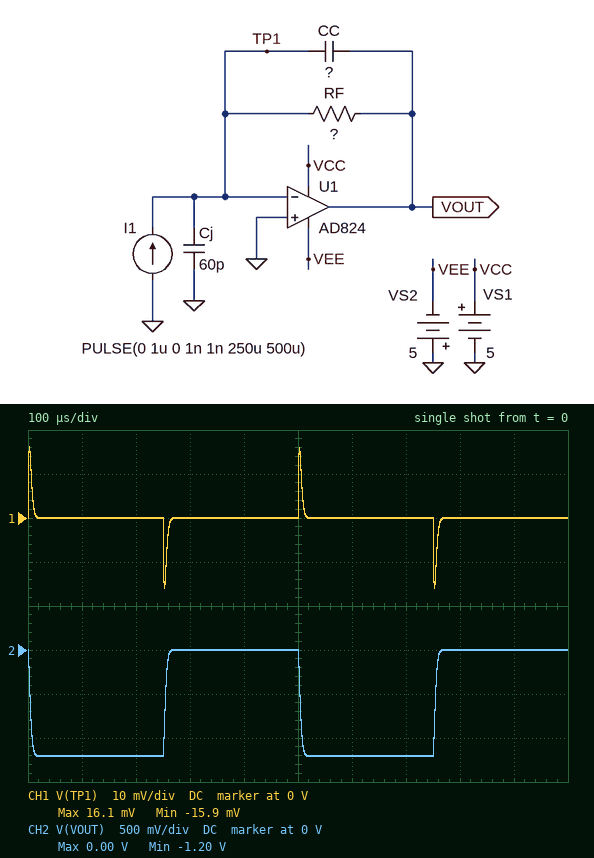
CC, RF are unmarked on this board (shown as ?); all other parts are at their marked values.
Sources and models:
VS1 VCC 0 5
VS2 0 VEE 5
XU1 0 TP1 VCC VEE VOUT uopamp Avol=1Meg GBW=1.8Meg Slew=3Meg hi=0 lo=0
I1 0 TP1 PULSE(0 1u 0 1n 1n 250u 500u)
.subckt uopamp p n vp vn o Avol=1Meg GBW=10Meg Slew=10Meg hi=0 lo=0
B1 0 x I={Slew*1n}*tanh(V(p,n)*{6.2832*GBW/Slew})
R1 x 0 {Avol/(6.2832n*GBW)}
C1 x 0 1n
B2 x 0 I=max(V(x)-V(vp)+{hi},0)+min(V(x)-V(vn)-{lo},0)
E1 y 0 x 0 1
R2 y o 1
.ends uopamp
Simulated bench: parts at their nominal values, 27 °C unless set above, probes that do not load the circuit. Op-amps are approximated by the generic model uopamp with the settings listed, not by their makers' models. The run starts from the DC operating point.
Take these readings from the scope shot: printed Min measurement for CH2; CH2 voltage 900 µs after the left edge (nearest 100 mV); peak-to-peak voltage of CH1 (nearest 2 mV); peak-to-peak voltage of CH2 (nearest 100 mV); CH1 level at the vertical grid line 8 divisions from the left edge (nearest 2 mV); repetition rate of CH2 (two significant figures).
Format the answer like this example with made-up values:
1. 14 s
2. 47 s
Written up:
1. -1.20 V
2. 0 V
3. 32 mV
4. 1.2 V
5. 0 V
6. 2.0 kHz
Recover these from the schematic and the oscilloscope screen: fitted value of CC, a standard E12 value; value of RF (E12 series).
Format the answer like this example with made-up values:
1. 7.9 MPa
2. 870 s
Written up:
1. 3.9 pF
2. 1.2 MΩ
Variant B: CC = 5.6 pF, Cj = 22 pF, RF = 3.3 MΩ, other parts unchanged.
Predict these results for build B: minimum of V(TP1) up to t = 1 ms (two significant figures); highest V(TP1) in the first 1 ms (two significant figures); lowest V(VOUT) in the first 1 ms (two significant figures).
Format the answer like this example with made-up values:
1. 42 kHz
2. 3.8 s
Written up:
1. -15 mV
2. 15 mV
3. -3.3 V
